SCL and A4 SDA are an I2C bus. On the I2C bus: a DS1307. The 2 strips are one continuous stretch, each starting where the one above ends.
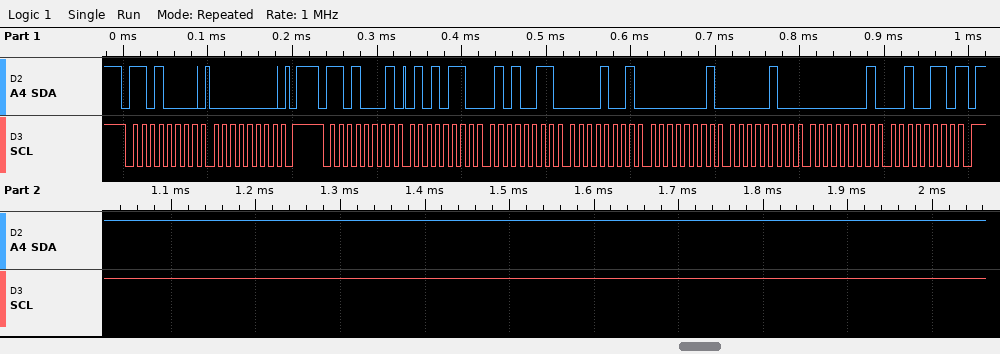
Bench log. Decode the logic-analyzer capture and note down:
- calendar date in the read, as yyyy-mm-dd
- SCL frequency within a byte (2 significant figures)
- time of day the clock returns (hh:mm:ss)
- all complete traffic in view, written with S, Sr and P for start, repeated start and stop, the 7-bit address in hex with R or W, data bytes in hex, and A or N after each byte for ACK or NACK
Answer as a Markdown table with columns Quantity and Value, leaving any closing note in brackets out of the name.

| Quantity | Value |
|---|---|
| calendar date in the read, as yyyy-mm-dd | 2026-01-04 |
| SCL frequency within a byte | 100 kHz |
| time of day the clock returns | 09:53:56 |
| all complete traffic in view, written with S, Sr and P for start, repeated start and stop, the 7-bit address in hex with R or W, data bytes in hex, and A or N after each byte for ACK or NACK | S 68W A 00 A P S 68R A 56 A 53 A 09 A 01 A 04 A 01 A 26 N P |
